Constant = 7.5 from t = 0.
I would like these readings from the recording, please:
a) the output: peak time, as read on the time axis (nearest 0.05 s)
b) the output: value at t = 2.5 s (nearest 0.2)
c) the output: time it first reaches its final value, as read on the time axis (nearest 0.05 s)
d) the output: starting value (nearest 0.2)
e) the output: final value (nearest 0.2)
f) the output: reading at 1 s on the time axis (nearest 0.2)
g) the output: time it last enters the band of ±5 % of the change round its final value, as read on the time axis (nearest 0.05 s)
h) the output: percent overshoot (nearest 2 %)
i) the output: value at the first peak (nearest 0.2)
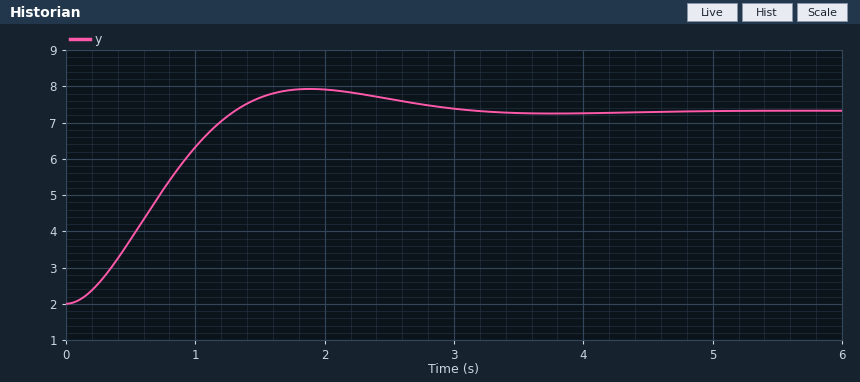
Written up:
1.90 s
7.6
1.30 s
2.0
7.4
6.4
2.60 s
12 %
8.0
